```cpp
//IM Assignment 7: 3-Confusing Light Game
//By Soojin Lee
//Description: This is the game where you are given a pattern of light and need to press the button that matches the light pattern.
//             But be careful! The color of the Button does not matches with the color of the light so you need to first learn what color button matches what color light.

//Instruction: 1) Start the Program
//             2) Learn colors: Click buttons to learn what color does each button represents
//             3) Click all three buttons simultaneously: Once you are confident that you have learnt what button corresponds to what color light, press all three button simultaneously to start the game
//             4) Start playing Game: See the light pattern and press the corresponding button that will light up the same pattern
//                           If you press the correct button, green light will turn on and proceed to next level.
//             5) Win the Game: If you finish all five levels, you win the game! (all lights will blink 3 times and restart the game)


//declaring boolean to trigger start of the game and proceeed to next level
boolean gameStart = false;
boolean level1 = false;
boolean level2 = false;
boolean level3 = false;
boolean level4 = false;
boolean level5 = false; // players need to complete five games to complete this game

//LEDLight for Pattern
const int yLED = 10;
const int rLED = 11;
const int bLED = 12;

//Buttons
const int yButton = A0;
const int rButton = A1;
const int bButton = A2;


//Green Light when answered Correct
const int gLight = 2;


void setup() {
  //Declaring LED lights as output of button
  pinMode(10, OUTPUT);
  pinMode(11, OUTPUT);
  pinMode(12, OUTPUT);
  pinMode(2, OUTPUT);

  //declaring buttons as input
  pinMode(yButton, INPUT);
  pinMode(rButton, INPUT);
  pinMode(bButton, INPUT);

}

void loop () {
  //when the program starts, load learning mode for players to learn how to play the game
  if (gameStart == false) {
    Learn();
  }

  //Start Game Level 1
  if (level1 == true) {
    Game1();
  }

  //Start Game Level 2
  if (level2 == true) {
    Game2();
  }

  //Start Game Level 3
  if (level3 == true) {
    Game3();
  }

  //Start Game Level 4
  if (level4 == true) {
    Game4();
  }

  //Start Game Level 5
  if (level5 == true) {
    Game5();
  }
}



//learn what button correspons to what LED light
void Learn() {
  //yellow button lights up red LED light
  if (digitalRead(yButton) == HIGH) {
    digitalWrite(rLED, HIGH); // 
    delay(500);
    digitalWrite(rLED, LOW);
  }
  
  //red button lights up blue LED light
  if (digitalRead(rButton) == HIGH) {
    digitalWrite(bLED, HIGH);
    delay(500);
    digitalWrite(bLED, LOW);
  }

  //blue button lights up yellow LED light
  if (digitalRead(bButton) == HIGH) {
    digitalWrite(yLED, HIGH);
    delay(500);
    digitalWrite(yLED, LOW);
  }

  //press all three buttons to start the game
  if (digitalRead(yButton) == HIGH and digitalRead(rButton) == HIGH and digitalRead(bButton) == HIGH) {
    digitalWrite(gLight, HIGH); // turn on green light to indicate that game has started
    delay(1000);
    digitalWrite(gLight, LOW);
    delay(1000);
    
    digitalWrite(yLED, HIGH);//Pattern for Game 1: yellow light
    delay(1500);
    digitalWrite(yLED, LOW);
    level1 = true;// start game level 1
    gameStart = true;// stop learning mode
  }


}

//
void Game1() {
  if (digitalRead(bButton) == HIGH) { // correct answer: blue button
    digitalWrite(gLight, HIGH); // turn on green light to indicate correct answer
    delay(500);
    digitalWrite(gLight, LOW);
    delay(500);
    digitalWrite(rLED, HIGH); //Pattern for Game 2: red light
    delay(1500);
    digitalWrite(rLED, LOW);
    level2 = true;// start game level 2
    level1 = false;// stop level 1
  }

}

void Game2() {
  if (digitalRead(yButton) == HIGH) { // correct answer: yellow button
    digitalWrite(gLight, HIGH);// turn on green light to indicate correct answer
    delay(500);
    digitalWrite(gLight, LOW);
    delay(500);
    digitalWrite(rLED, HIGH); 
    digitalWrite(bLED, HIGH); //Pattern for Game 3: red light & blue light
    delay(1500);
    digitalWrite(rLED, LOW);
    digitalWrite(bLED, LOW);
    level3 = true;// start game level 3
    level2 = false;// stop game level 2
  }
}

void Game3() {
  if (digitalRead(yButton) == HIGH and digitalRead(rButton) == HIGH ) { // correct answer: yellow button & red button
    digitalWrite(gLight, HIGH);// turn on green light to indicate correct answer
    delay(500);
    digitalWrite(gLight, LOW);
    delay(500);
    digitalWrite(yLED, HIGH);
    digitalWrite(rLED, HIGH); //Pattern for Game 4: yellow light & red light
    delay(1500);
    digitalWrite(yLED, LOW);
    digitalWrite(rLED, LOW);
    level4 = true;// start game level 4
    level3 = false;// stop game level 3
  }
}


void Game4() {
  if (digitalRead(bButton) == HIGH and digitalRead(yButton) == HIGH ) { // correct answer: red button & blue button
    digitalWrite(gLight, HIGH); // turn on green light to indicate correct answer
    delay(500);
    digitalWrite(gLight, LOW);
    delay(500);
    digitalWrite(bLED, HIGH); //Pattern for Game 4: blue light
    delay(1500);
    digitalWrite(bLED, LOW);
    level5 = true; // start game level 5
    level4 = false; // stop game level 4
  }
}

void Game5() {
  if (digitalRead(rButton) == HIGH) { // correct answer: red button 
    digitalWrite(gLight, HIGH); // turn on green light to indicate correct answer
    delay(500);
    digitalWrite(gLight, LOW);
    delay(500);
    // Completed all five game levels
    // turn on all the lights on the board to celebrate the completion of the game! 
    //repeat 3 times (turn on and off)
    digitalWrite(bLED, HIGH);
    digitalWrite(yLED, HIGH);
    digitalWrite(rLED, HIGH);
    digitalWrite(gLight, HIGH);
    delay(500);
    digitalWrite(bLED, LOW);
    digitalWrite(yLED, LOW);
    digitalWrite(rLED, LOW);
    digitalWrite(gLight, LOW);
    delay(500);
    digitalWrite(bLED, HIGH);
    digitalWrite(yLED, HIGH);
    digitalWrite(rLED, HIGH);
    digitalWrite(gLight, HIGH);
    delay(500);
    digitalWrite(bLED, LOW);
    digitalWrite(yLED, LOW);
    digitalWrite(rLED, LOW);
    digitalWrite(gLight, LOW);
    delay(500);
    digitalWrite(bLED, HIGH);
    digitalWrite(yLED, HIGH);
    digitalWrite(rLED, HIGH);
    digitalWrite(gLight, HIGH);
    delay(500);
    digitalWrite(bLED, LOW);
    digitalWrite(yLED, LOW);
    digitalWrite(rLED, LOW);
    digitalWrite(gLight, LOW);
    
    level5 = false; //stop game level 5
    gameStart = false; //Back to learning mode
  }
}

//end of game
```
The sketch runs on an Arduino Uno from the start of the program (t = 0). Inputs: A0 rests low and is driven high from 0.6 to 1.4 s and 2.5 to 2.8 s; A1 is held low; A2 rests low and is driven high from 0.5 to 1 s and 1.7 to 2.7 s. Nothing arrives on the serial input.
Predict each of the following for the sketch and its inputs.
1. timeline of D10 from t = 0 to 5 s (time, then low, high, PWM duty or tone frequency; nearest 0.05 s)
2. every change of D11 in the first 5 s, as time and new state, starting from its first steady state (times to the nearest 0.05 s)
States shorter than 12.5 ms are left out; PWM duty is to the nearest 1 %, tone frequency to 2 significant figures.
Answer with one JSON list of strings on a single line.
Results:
["0 s low; 0.5 s high; 1 s low; 1.7 s high; 2.7 s low", "0 s low; 1 s high; 1.5 s low; 2.7 s high; 3.2 s low"]
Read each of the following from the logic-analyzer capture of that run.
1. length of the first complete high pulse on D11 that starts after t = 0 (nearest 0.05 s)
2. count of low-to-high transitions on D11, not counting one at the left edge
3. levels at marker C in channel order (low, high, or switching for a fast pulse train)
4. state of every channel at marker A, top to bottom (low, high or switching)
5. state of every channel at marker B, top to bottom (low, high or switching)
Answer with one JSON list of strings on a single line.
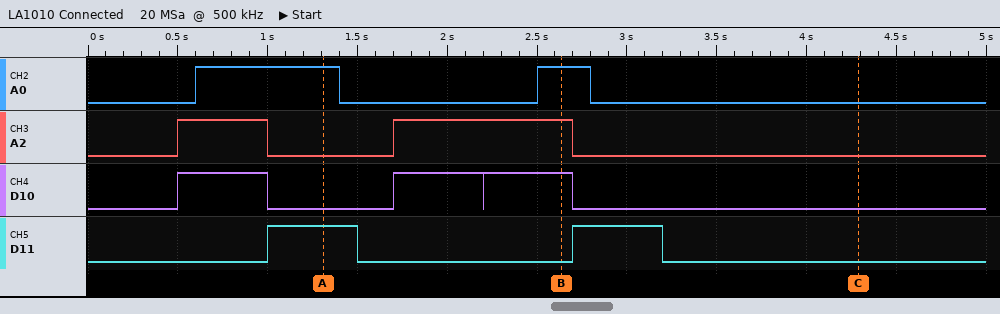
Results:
["0.50 s", "2", "A0 low, A2 low, D10 low, D11 low", "A0 high, A2 low, D10 low, D11 high", "A0 high, A2 high, D10 high, D11 low"]
